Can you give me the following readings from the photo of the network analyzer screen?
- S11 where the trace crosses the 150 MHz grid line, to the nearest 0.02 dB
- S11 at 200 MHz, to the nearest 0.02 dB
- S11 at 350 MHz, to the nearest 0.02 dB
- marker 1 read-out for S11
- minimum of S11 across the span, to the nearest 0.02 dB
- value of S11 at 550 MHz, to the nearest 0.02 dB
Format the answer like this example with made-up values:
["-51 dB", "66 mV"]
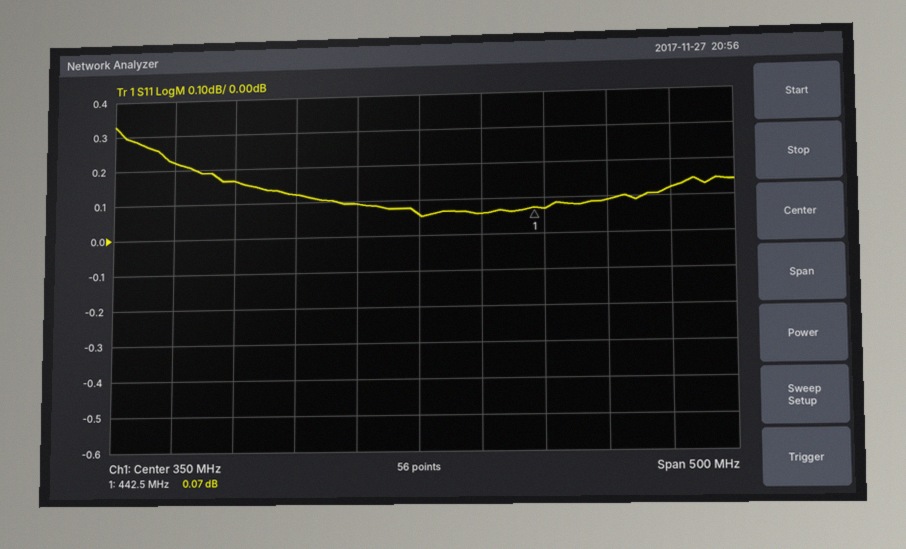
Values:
["0.22 dB", "0.16 dB", "0.06 dB", "0.07 dB", "0.06 dB", "0.12 dB"]
